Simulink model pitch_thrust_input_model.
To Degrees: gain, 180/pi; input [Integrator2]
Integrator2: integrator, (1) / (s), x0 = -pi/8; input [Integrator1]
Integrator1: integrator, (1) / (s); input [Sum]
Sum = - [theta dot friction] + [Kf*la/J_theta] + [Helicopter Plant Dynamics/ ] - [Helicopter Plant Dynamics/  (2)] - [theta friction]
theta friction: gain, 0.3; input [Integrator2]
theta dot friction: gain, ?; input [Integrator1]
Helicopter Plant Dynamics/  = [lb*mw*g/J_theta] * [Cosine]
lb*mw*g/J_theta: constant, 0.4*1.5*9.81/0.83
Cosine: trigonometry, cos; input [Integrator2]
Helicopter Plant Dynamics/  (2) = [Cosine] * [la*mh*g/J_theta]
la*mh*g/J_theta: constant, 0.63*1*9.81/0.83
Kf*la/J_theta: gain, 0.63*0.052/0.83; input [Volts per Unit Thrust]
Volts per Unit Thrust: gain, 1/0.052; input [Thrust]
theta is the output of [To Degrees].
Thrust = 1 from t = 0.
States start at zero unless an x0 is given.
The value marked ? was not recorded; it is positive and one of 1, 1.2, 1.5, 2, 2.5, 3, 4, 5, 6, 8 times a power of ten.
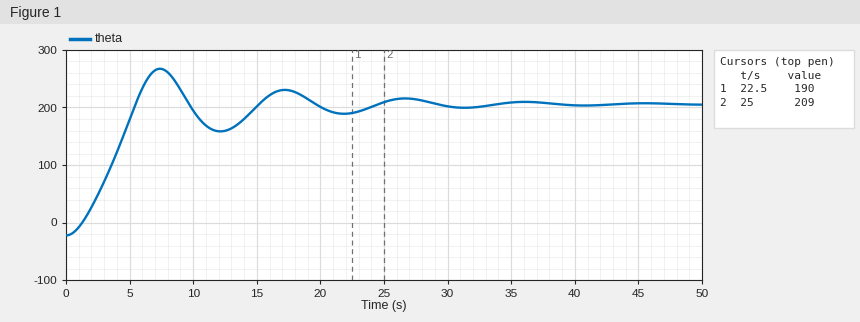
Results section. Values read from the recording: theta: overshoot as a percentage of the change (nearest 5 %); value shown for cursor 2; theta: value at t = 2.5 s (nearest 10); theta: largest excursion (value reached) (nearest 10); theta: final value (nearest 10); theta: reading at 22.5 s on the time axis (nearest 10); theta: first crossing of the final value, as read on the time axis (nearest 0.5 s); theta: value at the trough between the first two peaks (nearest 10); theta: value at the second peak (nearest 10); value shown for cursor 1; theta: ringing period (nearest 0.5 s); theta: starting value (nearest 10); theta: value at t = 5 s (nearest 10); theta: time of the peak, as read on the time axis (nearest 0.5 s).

25 %
209
50
270
210
190
5.5 s
160
230
190
10.0 s
-20
180
7.5 s
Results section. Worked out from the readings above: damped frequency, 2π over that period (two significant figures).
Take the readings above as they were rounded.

0.63 rad/s
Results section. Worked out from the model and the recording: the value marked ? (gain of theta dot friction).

0.2
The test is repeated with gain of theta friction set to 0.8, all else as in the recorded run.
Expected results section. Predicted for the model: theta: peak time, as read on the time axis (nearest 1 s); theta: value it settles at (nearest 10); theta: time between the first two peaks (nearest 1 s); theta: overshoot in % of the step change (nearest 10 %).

4 s
30
8 s
80 %
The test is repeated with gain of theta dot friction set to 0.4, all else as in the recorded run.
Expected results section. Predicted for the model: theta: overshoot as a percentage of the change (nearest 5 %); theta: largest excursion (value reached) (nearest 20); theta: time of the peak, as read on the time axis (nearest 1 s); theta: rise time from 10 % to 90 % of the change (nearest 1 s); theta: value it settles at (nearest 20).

15 %
240
9 s
5 s
200
